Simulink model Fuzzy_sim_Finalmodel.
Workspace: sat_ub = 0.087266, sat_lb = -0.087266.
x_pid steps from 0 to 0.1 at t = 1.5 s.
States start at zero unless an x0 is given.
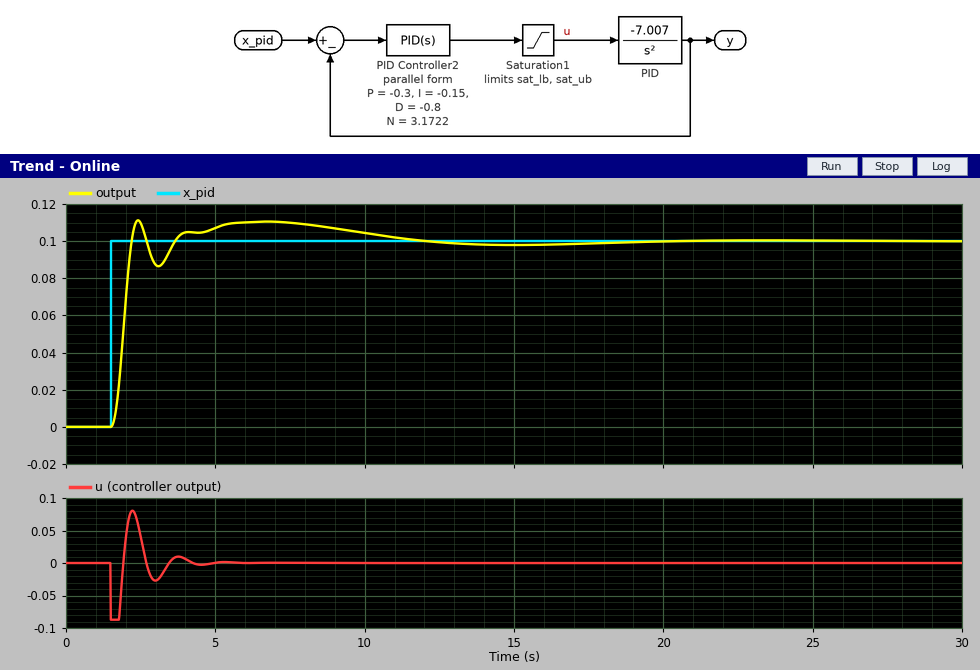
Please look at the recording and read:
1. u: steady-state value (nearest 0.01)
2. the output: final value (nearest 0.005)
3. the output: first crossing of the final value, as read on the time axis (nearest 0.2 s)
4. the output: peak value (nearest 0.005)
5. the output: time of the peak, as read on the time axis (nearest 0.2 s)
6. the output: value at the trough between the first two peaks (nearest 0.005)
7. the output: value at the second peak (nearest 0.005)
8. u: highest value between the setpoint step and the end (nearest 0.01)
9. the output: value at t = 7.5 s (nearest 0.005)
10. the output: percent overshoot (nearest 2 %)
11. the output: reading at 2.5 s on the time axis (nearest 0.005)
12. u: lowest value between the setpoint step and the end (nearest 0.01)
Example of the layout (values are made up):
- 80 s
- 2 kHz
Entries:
- 0.00
- 0.100
- 2.2 s
- 0.110
- 2.4 s
- 0.085
- 0.110
- 0.08
- 0.110
- 12 %
- 0.110
- -0.09
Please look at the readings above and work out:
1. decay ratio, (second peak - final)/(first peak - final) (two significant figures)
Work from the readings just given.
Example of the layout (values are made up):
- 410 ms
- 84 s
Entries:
- 1.0
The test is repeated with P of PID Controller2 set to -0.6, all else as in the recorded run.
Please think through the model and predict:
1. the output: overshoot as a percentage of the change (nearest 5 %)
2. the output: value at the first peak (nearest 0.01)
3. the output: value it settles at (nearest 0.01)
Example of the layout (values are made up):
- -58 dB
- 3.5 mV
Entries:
- 20 %
- 0.12
- 0.10
